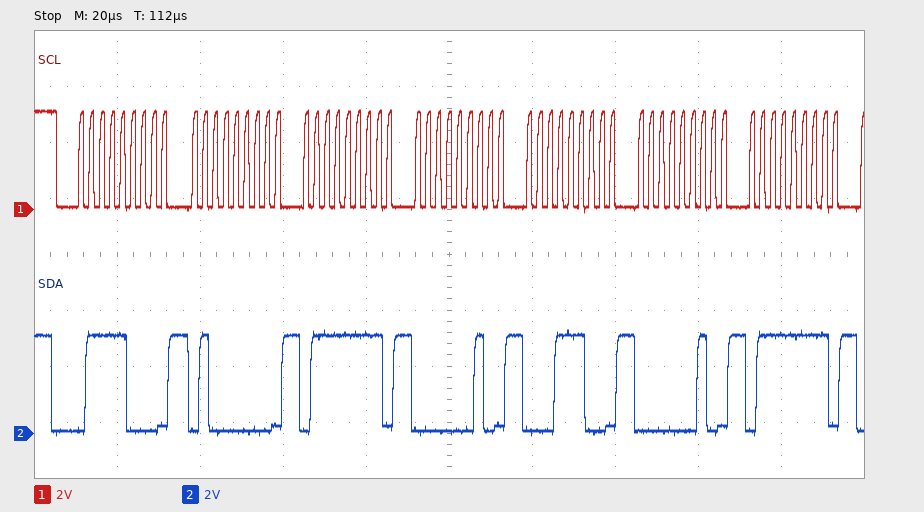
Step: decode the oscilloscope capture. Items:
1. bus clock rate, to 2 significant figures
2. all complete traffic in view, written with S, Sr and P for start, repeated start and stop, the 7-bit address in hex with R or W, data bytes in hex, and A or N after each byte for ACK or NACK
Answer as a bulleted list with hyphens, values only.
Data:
- 400 kHz
- S 3CW A 40 A 7F A 02 A 1C A 02 A 7F A
